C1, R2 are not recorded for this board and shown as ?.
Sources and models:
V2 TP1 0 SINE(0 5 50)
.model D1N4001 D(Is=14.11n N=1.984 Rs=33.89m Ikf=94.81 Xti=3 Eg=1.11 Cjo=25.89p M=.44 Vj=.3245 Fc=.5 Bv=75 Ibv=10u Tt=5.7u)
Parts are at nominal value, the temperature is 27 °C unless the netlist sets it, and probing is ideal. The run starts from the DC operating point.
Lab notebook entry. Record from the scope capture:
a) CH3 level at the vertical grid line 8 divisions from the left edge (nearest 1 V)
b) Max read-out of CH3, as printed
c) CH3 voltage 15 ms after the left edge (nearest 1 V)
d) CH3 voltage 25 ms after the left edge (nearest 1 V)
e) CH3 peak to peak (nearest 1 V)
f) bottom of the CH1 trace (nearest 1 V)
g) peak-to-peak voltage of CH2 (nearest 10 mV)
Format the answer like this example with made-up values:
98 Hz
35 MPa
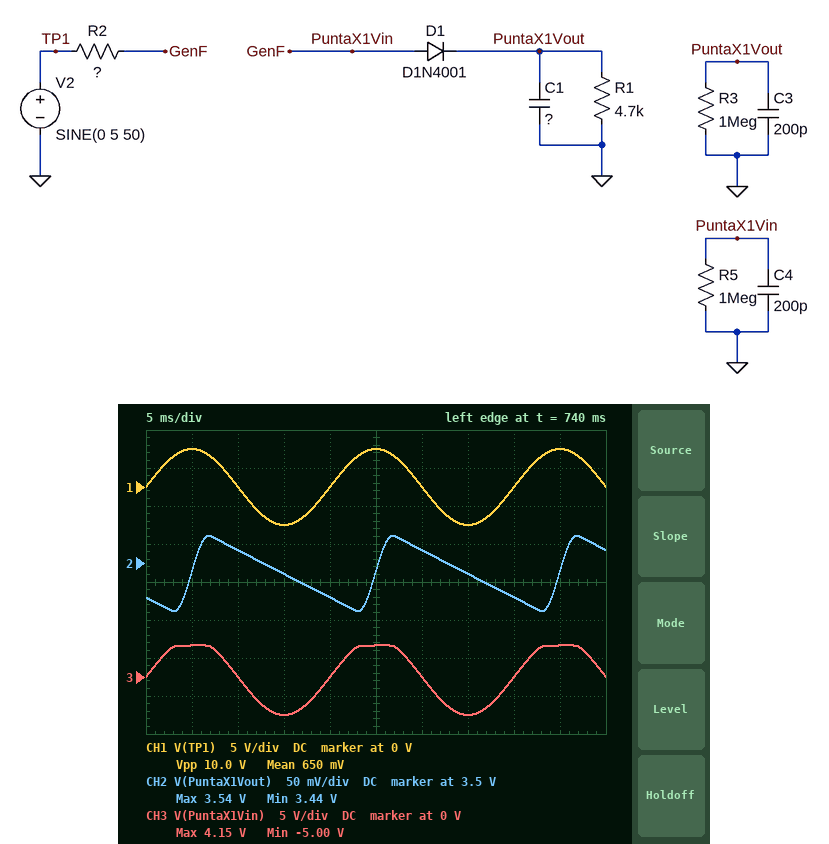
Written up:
0 V
4.15 V
-5 V
4 V
9 V
-5 V
100 mV
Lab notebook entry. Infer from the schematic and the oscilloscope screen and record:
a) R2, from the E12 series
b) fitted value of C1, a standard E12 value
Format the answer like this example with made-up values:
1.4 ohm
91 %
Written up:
150 Ω
120 µF
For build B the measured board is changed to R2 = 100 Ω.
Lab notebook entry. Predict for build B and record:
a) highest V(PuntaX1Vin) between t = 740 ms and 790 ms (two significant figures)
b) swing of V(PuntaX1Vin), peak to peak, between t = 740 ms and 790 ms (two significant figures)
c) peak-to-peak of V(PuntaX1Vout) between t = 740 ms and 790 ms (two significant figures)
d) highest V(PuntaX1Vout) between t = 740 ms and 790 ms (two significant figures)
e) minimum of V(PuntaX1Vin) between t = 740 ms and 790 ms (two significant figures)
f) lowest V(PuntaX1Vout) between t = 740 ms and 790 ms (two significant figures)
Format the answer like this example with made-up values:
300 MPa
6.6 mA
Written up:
4.4 V
9.4 V
110 mV
3.7 V
-5.0 V
3.6 V
